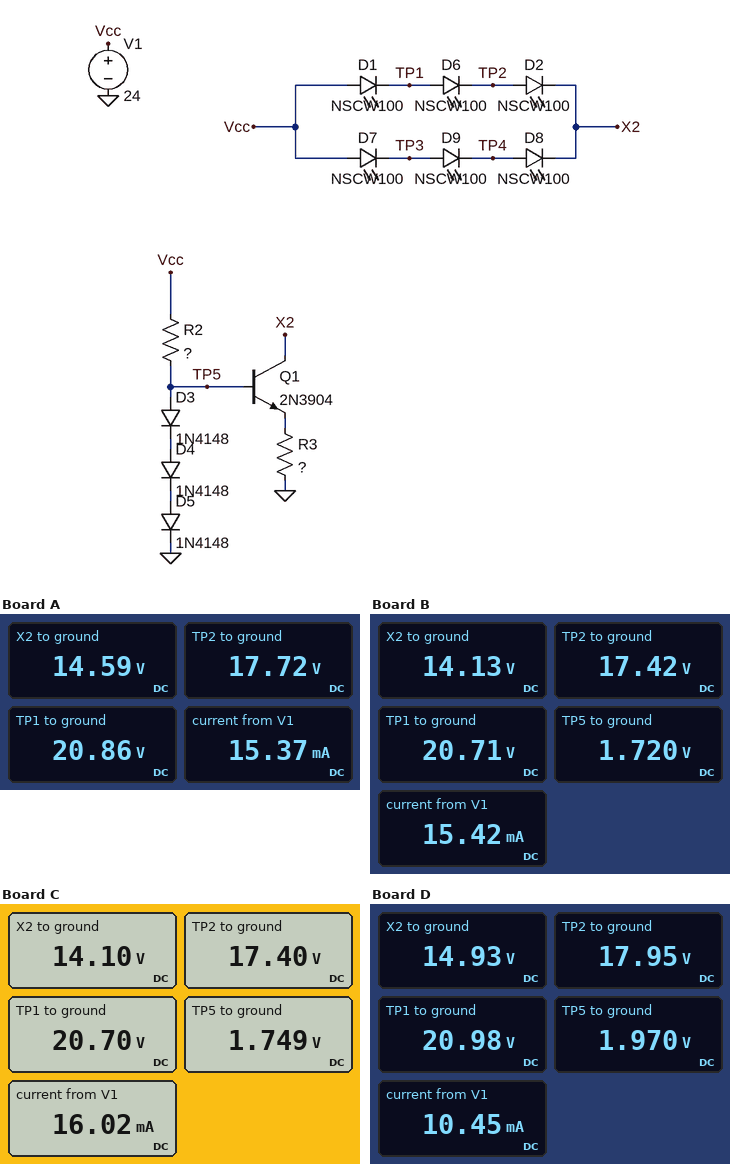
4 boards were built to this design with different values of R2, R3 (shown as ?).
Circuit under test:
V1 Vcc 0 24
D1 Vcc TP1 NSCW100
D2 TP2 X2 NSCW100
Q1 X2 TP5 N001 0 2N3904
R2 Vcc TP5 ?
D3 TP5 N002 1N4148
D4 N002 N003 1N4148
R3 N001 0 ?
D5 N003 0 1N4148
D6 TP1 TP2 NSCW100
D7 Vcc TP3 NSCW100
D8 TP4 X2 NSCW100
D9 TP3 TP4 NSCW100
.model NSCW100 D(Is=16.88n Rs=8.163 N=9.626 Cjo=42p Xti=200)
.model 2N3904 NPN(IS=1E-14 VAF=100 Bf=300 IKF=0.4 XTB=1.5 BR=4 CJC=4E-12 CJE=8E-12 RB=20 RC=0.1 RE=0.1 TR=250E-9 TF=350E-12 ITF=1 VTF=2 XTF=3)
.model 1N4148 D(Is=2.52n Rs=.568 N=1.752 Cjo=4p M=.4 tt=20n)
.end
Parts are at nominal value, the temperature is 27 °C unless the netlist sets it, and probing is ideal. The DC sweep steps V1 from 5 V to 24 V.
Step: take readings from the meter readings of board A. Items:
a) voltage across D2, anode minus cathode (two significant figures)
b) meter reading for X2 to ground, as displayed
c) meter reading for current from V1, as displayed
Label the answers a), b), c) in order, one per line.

a) 3.1 V
b) 14.59 V
c) 15.37 mA
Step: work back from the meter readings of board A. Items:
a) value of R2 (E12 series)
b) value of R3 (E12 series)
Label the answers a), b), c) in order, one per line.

a) 3.3 kΩ
b) 150 Ω
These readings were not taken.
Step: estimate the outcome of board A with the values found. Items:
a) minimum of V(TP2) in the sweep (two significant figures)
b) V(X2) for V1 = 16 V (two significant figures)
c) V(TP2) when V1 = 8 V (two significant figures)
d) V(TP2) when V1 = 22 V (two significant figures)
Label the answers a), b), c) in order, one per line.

a) 1.8 V
b) 6.6 V
c) 3.0 V
d) 16 V
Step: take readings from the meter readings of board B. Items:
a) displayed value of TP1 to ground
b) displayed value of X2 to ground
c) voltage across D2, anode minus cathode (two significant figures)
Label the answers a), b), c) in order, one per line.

a) 20.71 V
b) 14.13 V
c) 3.3 V
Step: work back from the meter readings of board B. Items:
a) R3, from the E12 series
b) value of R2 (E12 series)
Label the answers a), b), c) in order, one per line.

a) 68 Ω
b) 27 kΩ
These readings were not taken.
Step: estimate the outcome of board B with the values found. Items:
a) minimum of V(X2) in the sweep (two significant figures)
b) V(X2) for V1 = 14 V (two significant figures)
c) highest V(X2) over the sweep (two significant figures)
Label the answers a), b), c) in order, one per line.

a) 19 mV
b) 4.2 V
c) 14 V
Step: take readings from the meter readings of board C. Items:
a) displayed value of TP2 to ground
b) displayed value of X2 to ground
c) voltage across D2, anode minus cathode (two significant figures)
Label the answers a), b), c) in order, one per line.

a) 17.40 V
b) 14.10 V
c) 3.3 V
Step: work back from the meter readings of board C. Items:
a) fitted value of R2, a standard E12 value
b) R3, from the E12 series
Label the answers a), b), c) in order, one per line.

a) 22 kΩ
b) 68 Ω
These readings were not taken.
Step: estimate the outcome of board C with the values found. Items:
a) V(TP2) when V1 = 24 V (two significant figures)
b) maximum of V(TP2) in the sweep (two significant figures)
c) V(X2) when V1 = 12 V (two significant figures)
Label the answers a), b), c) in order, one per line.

a) 17 V
b) 17 V
c) 2.2 V
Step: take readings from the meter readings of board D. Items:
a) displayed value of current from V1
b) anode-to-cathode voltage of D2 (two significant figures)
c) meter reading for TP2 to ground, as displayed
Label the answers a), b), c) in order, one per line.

a) 10.45 mA
b) 3.0 V
c) 17.95 V
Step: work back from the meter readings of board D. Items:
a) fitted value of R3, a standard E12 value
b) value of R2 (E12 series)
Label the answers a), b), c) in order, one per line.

a) 220 Ω
b) 4.7 kΩ
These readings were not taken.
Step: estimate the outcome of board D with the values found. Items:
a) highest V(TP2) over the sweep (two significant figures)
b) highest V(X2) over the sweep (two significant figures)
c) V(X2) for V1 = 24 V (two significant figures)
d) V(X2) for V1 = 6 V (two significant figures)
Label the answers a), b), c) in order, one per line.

a) 18 V
b) 15 V
c) 15 V
d) 260 mV
